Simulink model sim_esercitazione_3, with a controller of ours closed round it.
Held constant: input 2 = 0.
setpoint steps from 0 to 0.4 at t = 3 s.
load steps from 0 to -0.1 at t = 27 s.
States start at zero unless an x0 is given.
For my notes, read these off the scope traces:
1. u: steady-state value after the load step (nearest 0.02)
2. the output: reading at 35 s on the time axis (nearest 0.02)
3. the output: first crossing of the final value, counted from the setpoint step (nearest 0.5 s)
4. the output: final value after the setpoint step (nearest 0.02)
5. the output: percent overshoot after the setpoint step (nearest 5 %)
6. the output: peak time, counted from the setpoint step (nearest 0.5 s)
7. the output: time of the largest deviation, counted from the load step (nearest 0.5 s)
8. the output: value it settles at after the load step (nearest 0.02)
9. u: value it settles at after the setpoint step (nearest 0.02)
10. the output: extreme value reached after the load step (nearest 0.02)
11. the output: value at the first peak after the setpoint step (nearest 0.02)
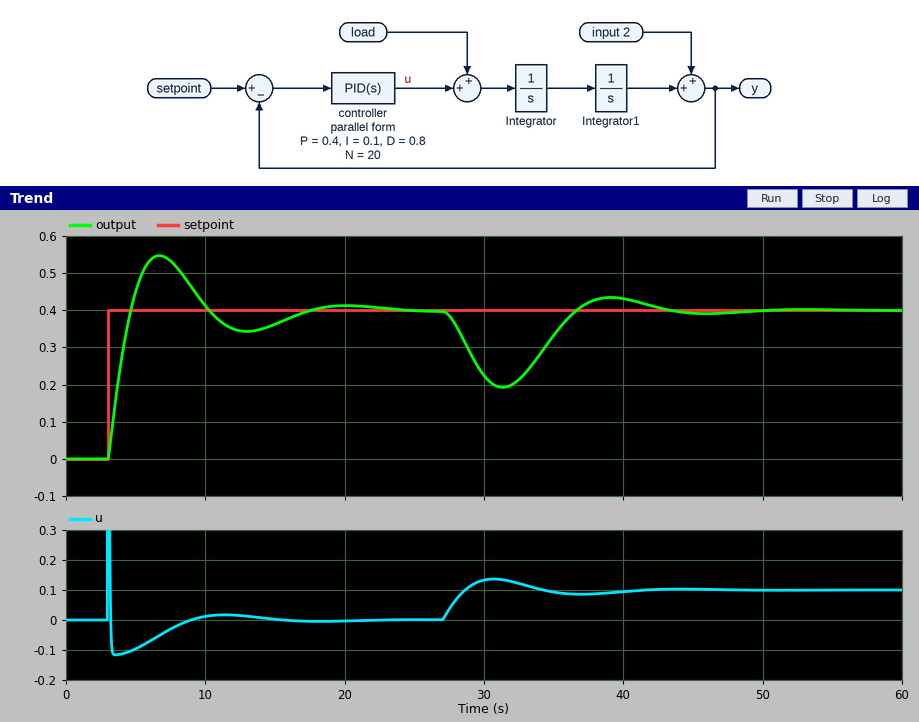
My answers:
0.10
0.34
1.5 s
0.40
35 %
3.5 s
4.5 s
0.40
0.00
0.20
0.54
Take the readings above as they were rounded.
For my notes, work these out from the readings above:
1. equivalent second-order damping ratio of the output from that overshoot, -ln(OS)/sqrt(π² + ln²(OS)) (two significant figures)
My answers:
0.32
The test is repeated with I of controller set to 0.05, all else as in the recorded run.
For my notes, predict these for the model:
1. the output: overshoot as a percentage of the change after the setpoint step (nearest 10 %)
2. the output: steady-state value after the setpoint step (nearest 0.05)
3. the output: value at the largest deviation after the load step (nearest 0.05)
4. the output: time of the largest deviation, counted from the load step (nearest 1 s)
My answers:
30 %
0.40
0.15
5 s
